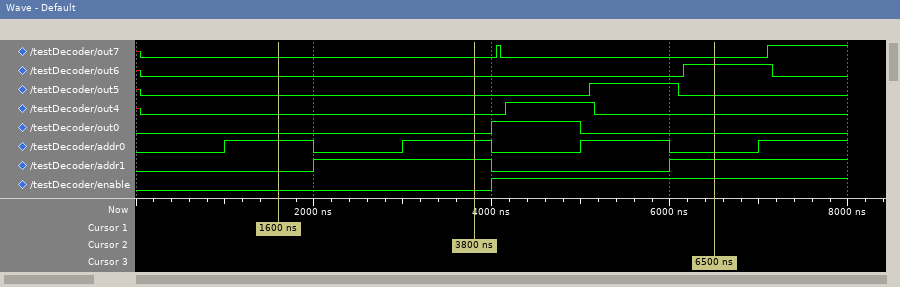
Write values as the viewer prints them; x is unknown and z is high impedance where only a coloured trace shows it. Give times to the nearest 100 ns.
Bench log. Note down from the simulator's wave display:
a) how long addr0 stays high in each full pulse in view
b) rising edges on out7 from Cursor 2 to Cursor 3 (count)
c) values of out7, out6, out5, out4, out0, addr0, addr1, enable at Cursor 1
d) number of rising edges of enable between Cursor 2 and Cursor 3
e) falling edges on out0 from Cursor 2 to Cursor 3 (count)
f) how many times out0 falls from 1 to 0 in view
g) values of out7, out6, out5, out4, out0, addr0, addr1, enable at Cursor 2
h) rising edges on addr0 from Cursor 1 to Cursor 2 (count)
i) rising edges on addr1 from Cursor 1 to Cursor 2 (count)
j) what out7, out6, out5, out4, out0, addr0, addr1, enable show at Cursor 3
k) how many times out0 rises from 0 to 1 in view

1000 ns, 1000 ns, 1000 ns
1
out7=0, out6=0, out5=0, out4=0, out0=0, addr0=1, addr1=0, enable=0
1
1
1
out7=0, out6=0, out5=0, out4=0, out0=0, addr0=1, addr1=1, enable=0
1
1
out7=0, out6=1, out5=0, out4=0, out0=0, addr0=0, addr1=1, enable=1
1
